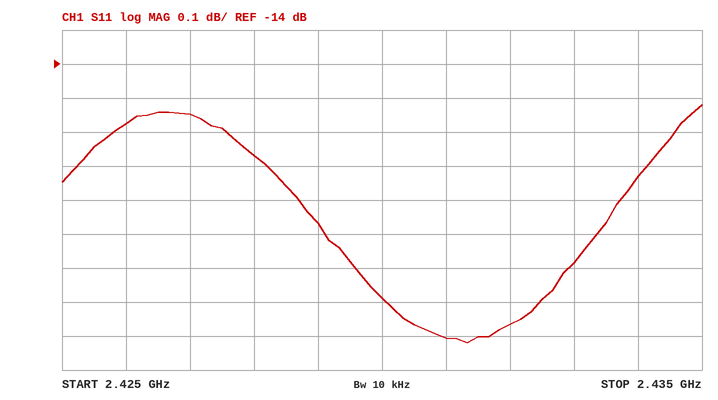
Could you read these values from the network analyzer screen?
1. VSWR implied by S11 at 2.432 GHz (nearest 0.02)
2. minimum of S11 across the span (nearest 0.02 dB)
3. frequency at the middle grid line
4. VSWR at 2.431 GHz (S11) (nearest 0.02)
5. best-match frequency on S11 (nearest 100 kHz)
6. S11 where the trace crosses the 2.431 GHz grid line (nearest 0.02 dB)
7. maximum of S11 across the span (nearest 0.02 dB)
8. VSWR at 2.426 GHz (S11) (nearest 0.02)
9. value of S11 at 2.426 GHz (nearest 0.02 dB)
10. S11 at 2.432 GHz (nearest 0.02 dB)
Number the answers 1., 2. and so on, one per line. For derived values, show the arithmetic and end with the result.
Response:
1. |Γ| = 10^(-14.76/20) = 0.1828; VSWR = (1 + 0.1828)/(1 − 0.1828) ≈ 1.45, so 1.44 to the nearest 0.02
2. -14.82 dB
3. 2.43 GHz
4. |Γ| = 10^(-14.8/20) = 0.1820; VSWR = (1 + 0.1820)/(1 − 0.1820) ≈ 1.44
5. 2.4313 GHz
6. -14.80 dB
7. -14.12 dB
8. |Γ| = 10^(-14.18/20) = 0.1954; VSWR = (1 + 0.1954)/(1 − 0.1954) ≈ 1.49, so 1.48 to the nearest 0.02
9. -14.18 dB
10. -14.76 dB
